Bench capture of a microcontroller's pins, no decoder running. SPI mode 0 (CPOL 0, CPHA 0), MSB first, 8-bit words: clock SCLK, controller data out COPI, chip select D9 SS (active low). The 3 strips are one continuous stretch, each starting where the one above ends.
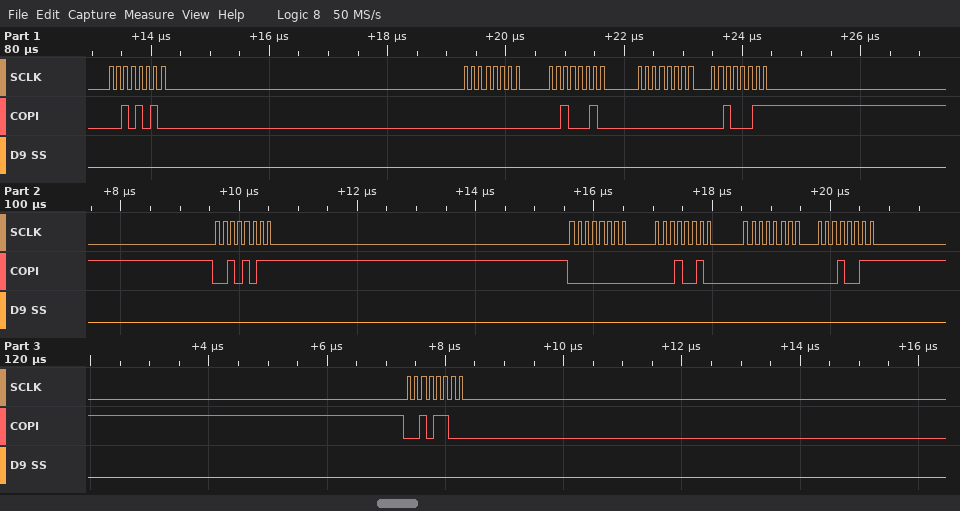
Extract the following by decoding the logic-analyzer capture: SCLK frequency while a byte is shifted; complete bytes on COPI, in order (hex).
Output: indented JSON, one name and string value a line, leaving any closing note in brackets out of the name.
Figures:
{
  "SCLK frequency while a byte is shifted": "8 MHz",
  "complete bytes on COPI, in order": "2A 00 22 00 23 2B 00 12 00 13 2C"
}
